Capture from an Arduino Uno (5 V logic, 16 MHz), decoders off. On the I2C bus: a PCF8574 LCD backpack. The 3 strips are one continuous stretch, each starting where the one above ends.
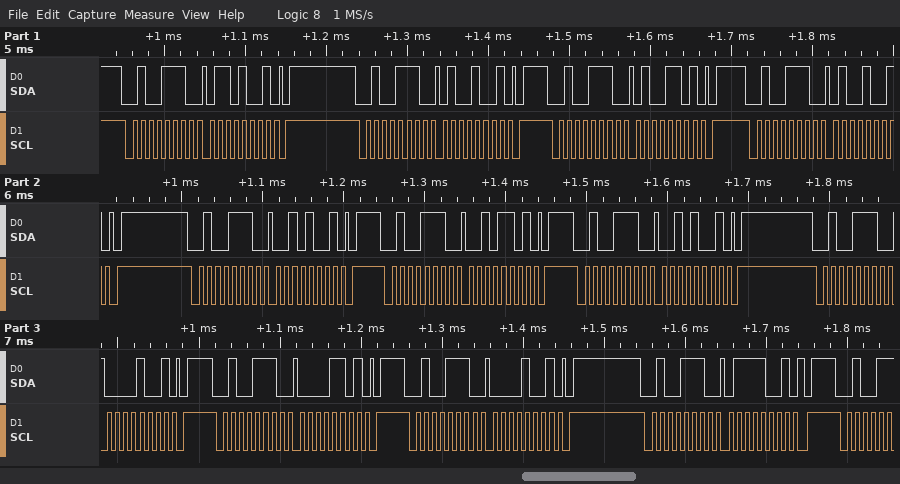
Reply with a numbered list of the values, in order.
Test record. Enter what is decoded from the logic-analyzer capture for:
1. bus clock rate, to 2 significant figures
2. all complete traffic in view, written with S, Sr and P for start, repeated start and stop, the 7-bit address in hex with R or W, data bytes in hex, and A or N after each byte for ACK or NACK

1. 100 kHz
2. S 27W A 69 A P S 27W A 49 A P S 27W A 4D A P S 27W A 49 A P S 27W A 29 A P S 27W A 2D A P S 27W A 29 A P S 27W A 09 A P S 27W A 0D A P S 27W A 09 A P S 27W A 79 A P
